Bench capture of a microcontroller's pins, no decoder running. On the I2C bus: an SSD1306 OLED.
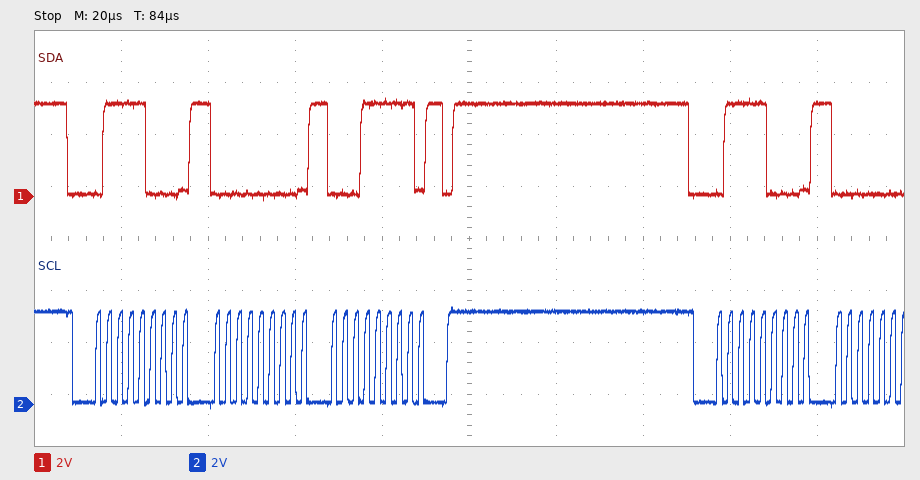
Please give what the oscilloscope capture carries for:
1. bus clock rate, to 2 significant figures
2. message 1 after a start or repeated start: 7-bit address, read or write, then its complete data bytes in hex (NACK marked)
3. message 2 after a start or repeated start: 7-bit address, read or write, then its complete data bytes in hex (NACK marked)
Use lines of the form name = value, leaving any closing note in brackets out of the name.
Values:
bus clock rate, to 2 significant figures = 400 kHz
message 1 after a start or repeated start: 7-bit address, read or write, then its complete data bytes in hex = 0x3C write: 00 1F
message 2 after a start or repeated start: 7-bit address, read or write, then its complete data bytes in hex = 0x3C write
